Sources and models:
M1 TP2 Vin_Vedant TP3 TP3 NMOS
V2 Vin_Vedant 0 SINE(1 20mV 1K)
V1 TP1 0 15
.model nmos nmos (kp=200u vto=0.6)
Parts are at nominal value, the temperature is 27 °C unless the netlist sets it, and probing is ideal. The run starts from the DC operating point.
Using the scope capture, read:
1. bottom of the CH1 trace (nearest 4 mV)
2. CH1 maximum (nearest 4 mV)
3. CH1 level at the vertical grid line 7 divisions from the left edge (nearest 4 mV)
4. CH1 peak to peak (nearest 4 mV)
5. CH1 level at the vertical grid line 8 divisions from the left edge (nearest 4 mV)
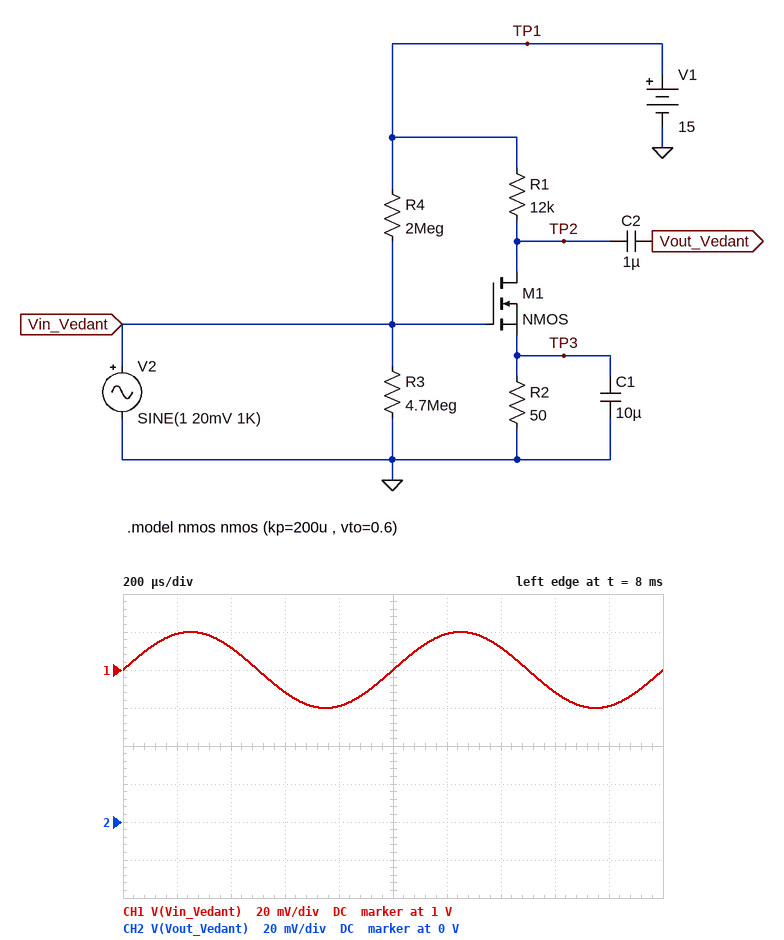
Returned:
980 mV
1.020 V
1.012 V
40 mV
988 mV
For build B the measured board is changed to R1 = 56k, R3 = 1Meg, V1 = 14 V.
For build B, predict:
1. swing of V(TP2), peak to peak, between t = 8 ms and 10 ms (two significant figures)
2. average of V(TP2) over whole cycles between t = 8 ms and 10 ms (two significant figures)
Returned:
180 mV
13 V
